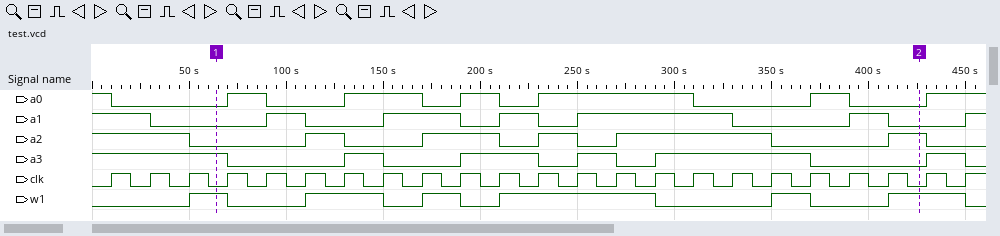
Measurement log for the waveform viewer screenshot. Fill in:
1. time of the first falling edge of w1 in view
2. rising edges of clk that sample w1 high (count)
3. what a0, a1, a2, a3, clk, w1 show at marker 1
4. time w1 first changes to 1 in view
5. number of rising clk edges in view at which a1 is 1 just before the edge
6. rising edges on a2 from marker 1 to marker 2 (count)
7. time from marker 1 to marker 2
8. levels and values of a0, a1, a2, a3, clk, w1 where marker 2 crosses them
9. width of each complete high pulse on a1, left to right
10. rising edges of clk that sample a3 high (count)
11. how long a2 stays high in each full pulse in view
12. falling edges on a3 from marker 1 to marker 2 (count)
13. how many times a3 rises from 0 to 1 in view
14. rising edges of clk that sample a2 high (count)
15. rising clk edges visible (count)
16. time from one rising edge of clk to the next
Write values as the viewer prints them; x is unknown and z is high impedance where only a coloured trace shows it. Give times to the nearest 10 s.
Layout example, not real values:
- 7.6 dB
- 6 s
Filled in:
- 70 s
- 11
- a0=0, a1=0, a2=0, a3=1, clk=0, w1=1
- 50 s
- 11
- 5
- 360 s
- a0=0, a1=0, a2=1, a3=0, clk=0, w1=1
- 20 s, 40 s, 20 s, 80 s, 20 s
- 13
- 20 s, 40 s, 20 s, 80 s, 20 s
- 5
- 5
- 12
- 23
- 20 s
